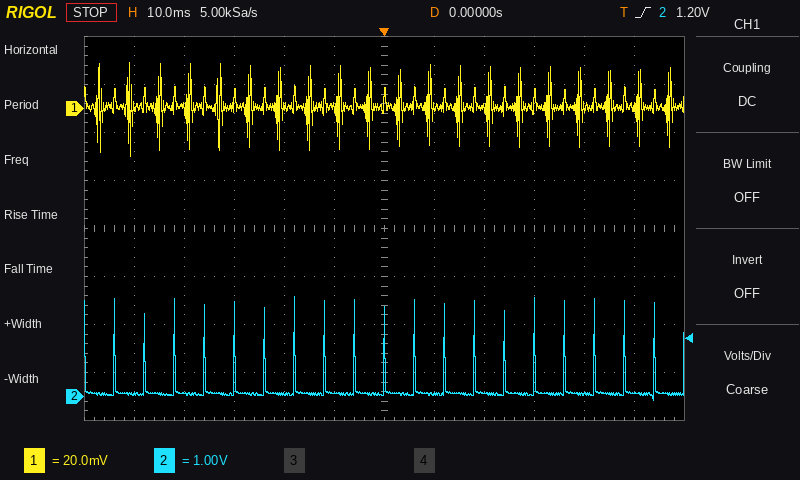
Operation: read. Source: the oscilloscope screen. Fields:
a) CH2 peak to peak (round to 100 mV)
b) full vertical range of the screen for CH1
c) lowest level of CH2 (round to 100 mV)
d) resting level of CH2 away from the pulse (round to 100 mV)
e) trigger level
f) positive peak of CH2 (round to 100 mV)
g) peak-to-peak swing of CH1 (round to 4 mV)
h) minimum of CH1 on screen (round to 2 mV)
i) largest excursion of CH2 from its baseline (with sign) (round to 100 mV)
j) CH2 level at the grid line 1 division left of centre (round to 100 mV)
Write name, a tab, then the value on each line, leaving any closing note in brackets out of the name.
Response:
CH2 peak to peak	2.2 V
full vertical range of the screen for CH1	160 mV
lowest level of CH2	-100 mV
resting level of CH2 away from the pulse	100 mV
trigger level	1.20 V
positive peak of CH2	2.1 V
peak-to-peak swing of CH1	40 mV
minimum of CH1 on screen	-20 mV
largest excursion of CH2 from its baseline (with sign)	+2.0 V
CH2 level at the grid line 1 division left of centre	100 mV
